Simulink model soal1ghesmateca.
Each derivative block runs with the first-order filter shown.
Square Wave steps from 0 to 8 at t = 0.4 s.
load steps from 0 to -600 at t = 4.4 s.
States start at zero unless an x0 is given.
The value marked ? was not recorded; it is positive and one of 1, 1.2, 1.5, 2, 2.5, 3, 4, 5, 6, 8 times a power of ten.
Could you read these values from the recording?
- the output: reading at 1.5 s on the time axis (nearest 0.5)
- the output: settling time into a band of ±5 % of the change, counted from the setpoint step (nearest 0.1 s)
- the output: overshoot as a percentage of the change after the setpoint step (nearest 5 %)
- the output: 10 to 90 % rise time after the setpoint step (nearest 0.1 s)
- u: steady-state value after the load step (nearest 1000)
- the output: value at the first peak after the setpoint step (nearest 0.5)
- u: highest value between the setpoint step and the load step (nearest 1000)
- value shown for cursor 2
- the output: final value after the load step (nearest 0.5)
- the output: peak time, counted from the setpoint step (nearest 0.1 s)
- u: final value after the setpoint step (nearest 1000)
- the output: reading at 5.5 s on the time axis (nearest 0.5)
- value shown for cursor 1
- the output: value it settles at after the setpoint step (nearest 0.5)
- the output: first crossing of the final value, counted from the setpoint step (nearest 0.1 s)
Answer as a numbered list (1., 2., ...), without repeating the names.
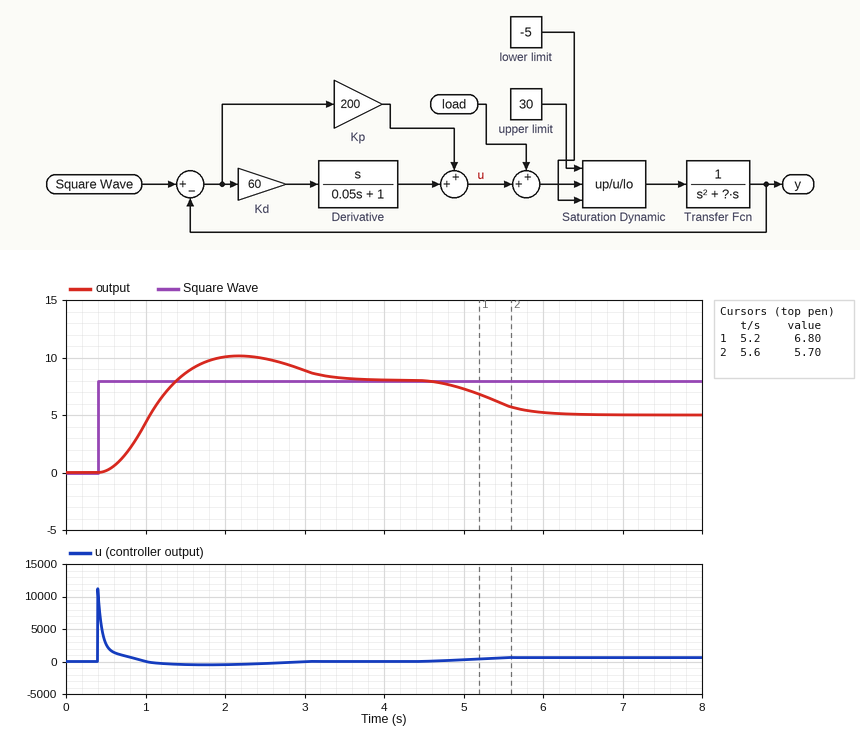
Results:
1. 8.5
2. 2.9 s
3. 25 %
4. 0.6 s
5. 1000
6. 10.0
7. 11000
8. 5.70
9. 5.0
10. 1.8 s
11. 0
12. 6.0
13. 6.80
14. 8.0
15. 1.0 s
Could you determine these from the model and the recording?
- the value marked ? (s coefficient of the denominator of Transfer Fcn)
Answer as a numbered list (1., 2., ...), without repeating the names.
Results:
1. 1.2
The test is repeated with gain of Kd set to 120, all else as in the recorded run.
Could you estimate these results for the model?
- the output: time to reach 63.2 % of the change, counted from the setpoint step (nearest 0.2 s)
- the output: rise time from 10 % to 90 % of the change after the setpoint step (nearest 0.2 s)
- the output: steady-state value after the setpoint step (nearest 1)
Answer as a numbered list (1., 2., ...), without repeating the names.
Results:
1. 0.8 s
2. 1.4 s
3. 8
